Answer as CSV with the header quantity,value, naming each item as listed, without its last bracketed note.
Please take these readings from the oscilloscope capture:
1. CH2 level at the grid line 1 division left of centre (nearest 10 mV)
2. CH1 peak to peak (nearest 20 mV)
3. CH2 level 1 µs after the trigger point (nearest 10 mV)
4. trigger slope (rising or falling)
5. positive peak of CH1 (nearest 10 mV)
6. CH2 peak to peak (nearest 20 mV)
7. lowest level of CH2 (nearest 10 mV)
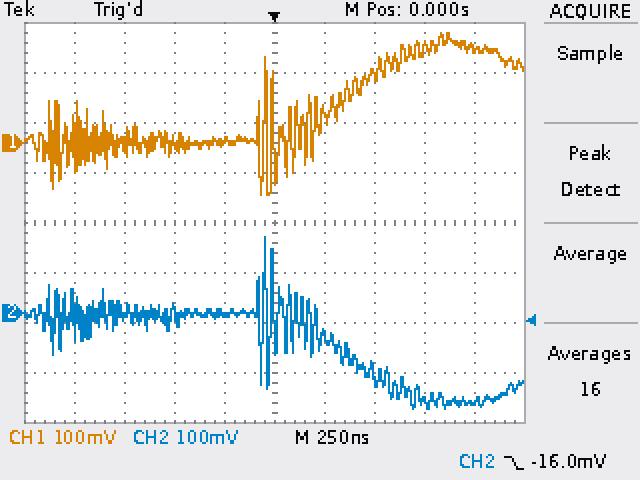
quantity,value
CH2 level at the grid line 1 division left of centre,0 mV
CH1 peak to peak,320 mV
CH2 level 1 µs after the trigger point,-180 mV
trigger slope,falling
positive peak of CH1,220 mV
CH2 peak to peak,340 mV
lowest level of CH2,-190 mV
